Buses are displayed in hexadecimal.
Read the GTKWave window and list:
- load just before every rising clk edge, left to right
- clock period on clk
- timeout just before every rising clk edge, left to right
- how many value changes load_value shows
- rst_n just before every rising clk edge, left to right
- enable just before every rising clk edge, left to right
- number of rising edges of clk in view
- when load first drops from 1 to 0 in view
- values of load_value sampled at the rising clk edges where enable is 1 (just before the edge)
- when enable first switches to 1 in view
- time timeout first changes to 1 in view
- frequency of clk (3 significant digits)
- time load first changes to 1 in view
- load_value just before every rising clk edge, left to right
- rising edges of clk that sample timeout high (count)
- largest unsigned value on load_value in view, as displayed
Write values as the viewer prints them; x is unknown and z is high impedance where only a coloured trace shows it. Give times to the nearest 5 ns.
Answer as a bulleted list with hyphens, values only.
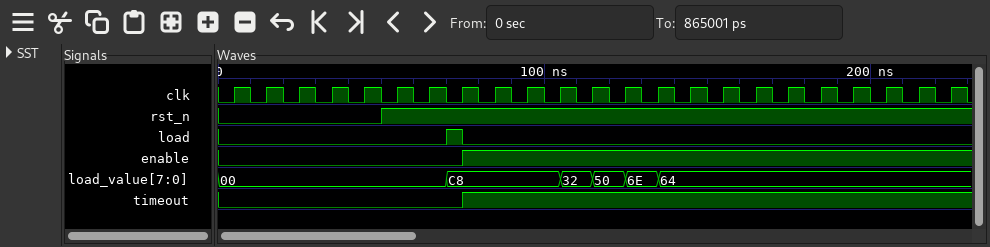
- 0 0 0 0 0 0 0 1 0 0 0 0 0 0 0 0 0 0 0 0 0 0 0
- 10 ns
- 0 0 0 0 0 0 0 0 1 1 1 1 1 1 1 1 1 1 1 1 1 1 1
- 5
- 0 0 0 0 0 1 1 1 1 1 1 1 1 1 1 1 1 1 1 1 1 1 1
- 0 0 0 0 0 0 0 0 1 1 1 1 1 1 1 1 1 1 1 1 1 1 1
- 23
- 75 ns
- C8, C8, C8, 32, 50, 6E, 64, 64, 64, 64, 64, 64, 64, 64, 64
- 75 ns
- 75 ns
- 100 MHz
- 70 ns
- 00, 00, 00, 00, 00, 00, 00, C8, C8, C8, C8, 32, 50, 6E, 64, 64, 64, 64, 64, 64, 64, 64, 64
- 15
- C8
